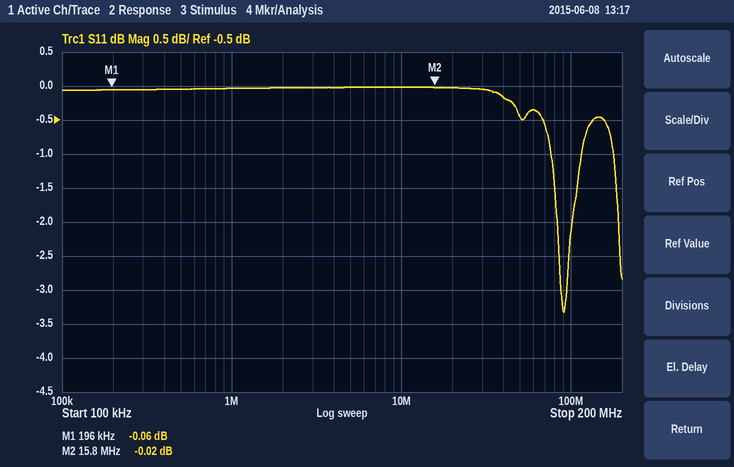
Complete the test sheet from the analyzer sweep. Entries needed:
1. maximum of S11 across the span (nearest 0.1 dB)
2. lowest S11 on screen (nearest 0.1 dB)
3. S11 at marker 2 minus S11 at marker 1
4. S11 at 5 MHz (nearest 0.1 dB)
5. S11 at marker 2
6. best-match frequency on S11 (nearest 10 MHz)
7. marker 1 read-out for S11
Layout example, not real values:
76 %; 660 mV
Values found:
0.0 dB; -3.3 dB; 0.04 dB; 0.0 dB; -0.02 dB; 90 MHz; -0.06 dB
